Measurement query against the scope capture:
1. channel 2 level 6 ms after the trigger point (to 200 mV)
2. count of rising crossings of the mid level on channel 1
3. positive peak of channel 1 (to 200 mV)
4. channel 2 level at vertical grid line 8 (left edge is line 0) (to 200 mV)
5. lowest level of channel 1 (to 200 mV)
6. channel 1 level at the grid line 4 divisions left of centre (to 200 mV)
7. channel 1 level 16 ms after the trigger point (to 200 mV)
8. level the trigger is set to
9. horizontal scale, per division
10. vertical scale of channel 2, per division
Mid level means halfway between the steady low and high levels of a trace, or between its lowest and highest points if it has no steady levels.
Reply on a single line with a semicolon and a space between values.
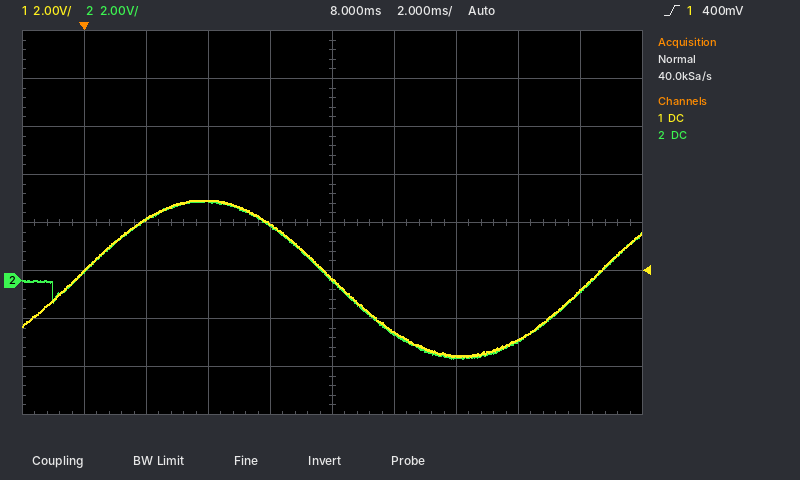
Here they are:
2.2 V; 2; 3.4 V; -2.6 V; -3.2 V; 400 mV; -400 mV; 400 mV; 2 ms; 2 V
